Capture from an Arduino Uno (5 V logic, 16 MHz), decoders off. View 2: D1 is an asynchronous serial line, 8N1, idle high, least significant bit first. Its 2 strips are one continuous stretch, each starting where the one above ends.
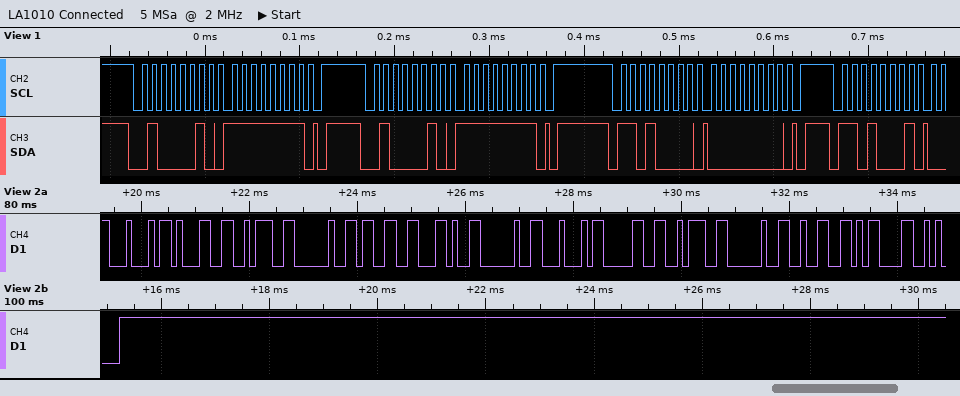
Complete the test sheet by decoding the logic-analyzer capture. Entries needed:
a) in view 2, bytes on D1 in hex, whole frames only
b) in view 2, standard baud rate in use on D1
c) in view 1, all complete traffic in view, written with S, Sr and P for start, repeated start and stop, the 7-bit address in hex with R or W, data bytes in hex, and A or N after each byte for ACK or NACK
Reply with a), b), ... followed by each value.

a) 44 31 3A 20 33 2C 20 44 30 3A 20 32 0D 0A
b) 9600 baud
c) S 21W A FF A P S 21W A FF A P S 68W A 00 A P S 68R A
